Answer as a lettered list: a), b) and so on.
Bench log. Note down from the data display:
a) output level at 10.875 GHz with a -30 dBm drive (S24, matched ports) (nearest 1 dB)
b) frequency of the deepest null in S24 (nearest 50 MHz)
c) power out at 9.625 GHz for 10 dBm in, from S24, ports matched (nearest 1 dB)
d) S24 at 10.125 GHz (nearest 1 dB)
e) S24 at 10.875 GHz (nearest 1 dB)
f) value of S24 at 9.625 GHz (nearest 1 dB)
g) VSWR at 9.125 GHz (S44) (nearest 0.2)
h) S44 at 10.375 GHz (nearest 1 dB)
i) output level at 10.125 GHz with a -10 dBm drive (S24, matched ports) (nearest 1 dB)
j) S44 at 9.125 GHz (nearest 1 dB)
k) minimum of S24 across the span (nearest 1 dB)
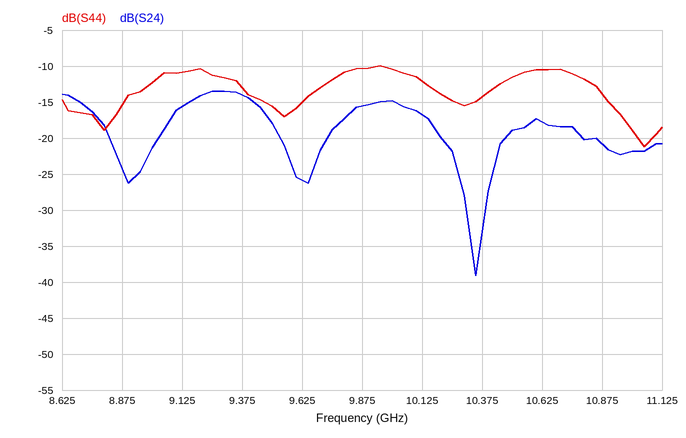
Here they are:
a) -51 dBm
b) 10.35 GHz
c) -16 dBm
d) -17 dB
e) -21 dB
f) -26 dB
g) 1.8
h) -14 dB
i) -27 dBm
j) -11 dB
k) -39 dB
